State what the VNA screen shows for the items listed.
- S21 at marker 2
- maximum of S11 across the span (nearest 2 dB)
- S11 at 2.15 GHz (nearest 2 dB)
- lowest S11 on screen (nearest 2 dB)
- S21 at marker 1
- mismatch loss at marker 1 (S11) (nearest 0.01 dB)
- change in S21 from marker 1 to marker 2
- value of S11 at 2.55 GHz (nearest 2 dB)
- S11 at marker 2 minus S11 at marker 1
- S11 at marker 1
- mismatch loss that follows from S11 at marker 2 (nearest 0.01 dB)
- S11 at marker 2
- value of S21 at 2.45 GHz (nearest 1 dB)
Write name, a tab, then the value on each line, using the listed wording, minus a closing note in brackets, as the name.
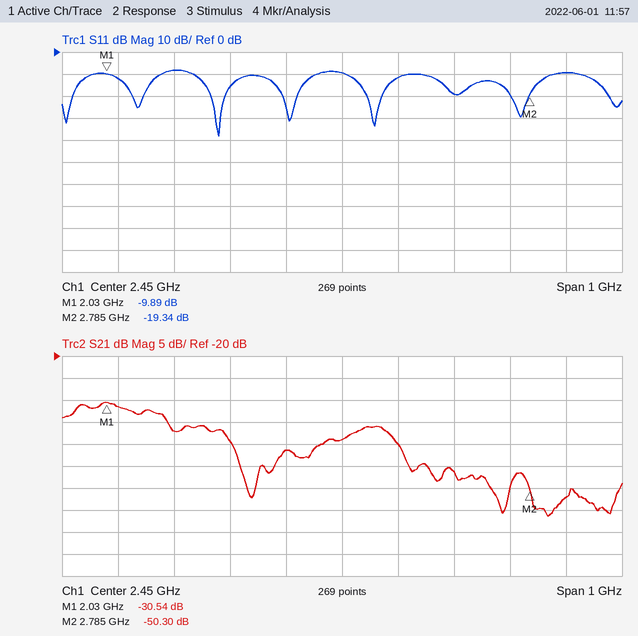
S21 at marker 2	-50.30 dB
maximum of S11 across the span	-8 dB
S11 at 2.15 GHz	-8 dB
lowest S11 on screen	-38 dB
S21 at marker 1	-30.54 dB
mismatch loss at marker 1 (S11)	0.47 dB
change in S21 from marker 1 to marker 2	-19.76 dB
value of S11 at 2.55 GHz	-12 dB
S11 at marker 2 minus S11 at marker 1	-9.45 dB
S11 at marker 1	-9.89 dB
mismatch loss that follows from S11 at marker 2	0.05 dB
S11 at marker 2	-19.34 dB
value of S21 at 2.45 GHz	-39 dB
